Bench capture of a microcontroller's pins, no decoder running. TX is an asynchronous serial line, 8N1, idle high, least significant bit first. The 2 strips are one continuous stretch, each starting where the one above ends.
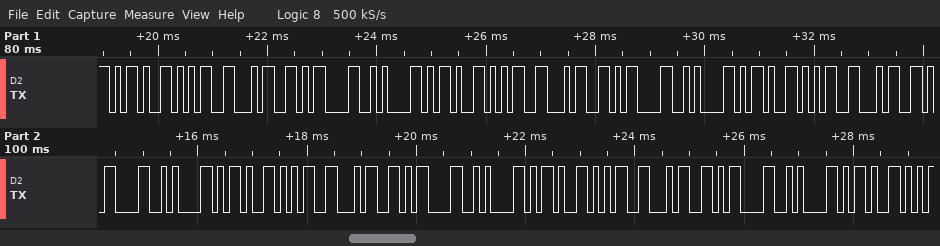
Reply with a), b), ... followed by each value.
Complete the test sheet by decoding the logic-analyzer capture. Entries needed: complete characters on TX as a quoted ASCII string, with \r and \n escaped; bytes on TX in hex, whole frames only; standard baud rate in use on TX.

a) "-54\r\n-54\r\n-54\r\n-54\r\n-54\r\n-"
b) 2D 35 34 0D 0A 2D 35 34 0D 0A 2D 35 34 0D 0A 2D 35 34 0D 0A 2D 35 34 0D 0A 2D
c) 9600 baud
